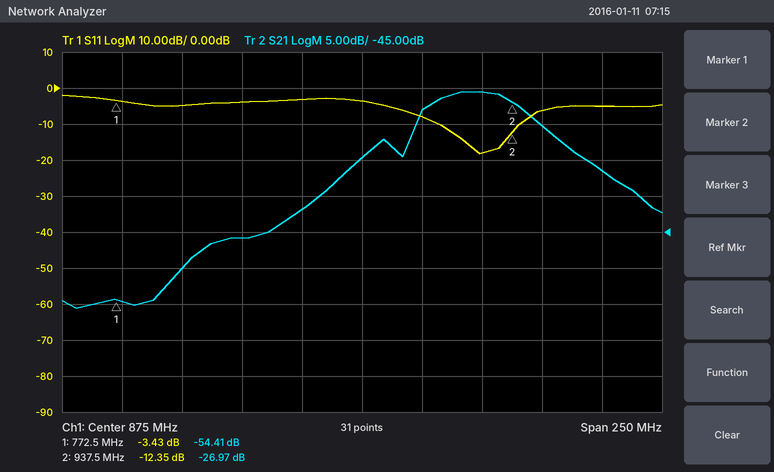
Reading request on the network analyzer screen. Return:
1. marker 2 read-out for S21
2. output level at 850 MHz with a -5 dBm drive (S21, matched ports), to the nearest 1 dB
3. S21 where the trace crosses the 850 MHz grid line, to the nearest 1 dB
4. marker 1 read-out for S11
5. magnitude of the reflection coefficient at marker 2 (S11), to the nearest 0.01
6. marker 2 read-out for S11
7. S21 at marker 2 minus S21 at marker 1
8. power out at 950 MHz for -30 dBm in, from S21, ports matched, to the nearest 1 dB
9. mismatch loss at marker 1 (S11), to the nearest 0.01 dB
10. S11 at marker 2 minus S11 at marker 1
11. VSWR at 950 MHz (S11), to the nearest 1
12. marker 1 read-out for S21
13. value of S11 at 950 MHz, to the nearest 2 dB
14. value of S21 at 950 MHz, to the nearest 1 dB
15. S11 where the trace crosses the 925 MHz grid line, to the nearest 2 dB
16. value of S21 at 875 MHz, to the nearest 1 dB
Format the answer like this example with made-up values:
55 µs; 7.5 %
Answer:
-26.97 dB; -47 dBm; -42 dB; -3.43 dB; 0.24; -12.35 dB; 27.44 dB; -60 dBm; 2.63 dB; -8.92 dB; 3; -54.41 dB; -6 dB; -30 dB; -18 dB; -35 dB
